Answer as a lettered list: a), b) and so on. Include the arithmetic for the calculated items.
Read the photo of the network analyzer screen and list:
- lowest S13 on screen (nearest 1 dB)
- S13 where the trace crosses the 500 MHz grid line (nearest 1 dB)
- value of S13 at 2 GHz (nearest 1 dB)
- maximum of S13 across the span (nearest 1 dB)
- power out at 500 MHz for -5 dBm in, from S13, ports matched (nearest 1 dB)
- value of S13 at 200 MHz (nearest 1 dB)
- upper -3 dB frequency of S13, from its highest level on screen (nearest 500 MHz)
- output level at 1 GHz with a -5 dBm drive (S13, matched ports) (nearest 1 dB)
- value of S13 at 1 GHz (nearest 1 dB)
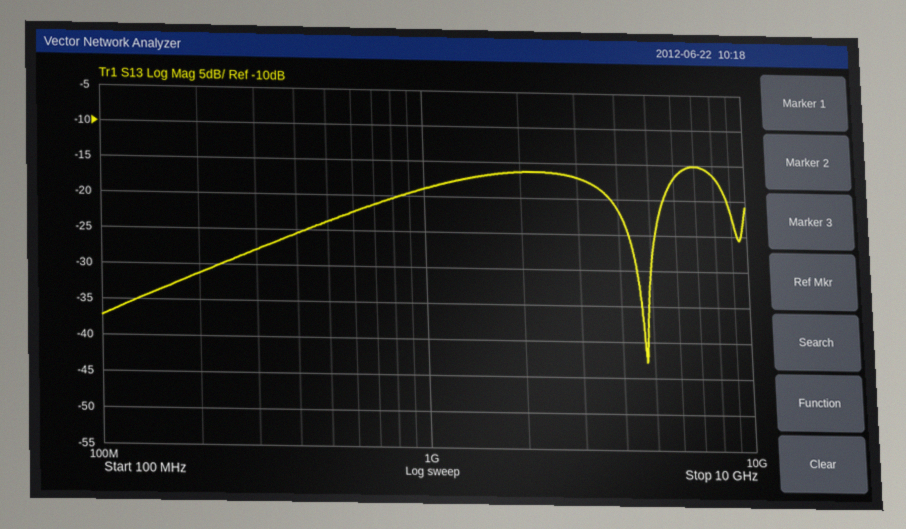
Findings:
a) -43 dB
b) -24 dB
c) -16 dB
d) -15 dB
e) -5 dBm + (-24 dB) = -29 dBm
f) -31 dB
g) 8.5 GHz
h) -5 dBm + (-19 dB) = -24 dBm
i) -19 dB
